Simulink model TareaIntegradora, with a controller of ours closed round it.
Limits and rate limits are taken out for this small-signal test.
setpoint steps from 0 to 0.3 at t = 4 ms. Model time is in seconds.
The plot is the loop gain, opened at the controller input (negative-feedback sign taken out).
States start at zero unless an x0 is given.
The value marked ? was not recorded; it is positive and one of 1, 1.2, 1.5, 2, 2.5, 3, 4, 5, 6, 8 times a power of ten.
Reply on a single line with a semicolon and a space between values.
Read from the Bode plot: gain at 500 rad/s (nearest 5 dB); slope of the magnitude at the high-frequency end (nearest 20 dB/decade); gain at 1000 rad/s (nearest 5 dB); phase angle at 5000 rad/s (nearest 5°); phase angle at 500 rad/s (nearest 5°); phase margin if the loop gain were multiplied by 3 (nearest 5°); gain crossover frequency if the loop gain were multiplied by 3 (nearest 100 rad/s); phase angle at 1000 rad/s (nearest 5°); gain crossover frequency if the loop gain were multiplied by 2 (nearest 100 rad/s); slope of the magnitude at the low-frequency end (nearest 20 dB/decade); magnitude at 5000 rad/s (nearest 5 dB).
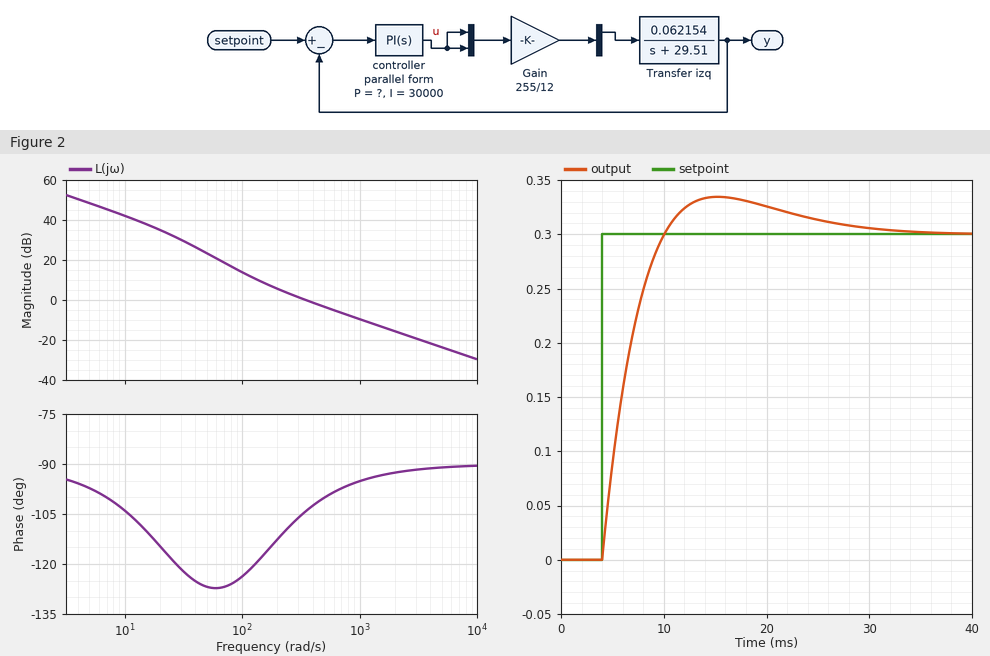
-5 dB; -20 dB/decade; -10 dB; -90°; -100°; 85°; 1000 rad/s; -95°; 700 rad/s; -20 dB/decade; -25 dB
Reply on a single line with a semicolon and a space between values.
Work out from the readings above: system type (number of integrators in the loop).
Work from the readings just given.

1
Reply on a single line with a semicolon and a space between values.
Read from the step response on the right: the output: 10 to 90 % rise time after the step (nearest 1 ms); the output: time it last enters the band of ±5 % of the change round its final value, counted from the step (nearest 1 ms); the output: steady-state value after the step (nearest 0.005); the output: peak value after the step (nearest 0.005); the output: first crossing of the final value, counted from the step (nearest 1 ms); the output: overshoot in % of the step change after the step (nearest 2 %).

4 ms; 20 ms; 0.300; 0.335; 6 ms; 12 %
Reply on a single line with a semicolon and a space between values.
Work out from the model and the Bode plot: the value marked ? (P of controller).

250
